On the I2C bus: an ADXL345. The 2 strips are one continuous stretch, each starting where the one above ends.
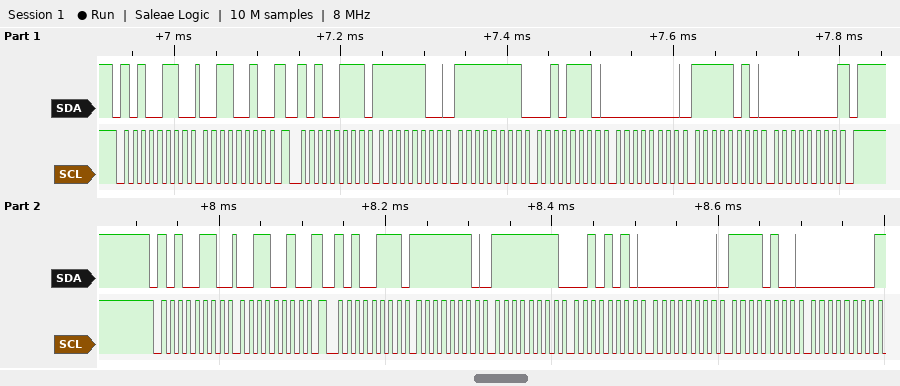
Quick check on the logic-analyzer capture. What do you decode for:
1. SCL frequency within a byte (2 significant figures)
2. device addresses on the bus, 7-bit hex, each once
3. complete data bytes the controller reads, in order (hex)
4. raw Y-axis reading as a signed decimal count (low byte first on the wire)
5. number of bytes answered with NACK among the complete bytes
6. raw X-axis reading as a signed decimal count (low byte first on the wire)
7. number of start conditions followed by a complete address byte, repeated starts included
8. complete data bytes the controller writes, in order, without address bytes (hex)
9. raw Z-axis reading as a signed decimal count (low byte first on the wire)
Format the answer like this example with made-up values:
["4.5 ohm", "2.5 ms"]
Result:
["100 kHz", "0x53", "FC FF 2E 00 FA 00 FE FF 2A 00 F4 00", "46", "2", "-4", "4", "32 32", "250"]
